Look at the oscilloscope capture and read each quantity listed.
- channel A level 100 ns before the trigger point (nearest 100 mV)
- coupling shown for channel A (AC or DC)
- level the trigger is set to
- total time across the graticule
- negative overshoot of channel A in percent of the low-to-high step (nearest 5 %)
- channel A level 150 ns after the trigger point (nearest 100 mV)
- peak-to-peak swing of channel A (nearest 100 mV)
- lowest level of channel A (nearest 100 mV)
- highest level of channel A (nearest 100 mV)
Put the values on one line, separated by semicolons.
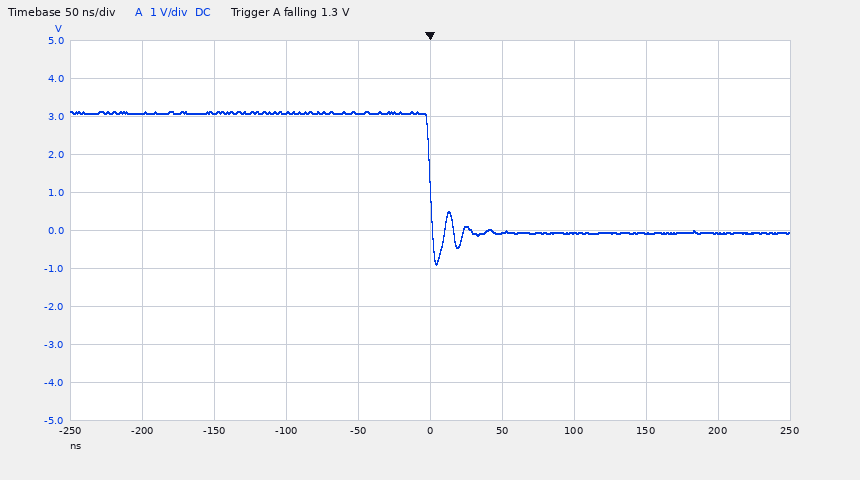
3.1 V; DC; 1.3 V; 500 ns; 25 %; -100 mV; 4.0 V; -900 mV; 3.1 V
